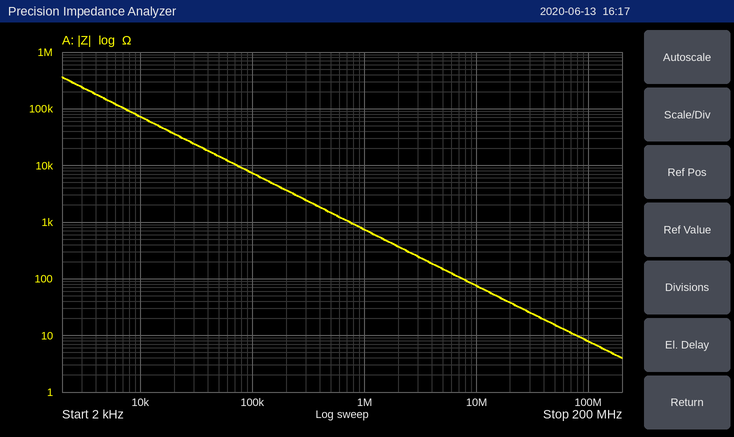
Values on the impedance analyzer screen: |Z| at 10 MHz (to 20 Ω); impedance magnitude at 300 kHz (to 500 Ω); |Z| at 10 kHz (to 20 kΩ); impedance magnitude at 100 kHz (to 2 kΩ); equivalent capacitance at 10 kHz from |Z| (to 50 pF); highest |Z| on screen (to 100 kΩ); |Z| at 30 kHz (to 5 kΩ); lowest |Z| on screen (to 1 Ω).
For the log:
80 Ω
2.5 kΩ
80 kΩ
8 kΩ
200 pF
400 kΩ
25 kΩ
4 Ω
